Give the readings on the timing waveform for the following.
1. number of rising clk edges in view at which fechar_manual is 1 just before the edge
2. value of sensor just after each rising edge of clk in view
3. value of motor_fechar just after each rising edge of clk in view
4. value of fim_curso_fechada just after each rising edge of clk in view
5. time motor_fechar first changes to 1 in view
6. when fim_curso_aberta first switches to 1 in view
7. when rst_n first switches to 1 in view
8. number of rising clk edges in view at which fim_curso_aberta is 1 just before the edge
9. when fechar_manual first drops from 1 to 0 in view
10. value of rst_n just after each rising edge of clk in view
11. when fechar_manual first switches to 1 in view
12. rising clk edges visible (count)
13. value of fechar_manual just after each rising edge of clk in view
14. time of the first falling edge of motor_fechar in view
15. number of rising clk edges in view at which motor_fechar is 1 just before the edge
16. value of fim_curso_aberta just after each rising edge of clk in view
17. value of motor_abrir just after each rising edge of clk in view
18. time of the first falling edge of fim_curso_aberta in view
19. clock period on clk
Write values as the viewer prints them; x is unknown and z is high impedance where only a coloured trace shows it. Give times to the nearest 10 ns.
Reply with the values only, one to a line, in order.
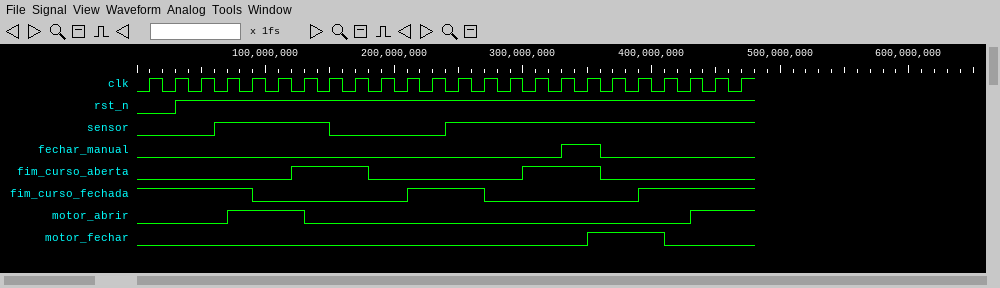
1
0 0 0 1 1 1 1 0 0 0 0 0 1 1 1 1 1 1 1 1 1 1 1 1
0 0 0 0 0 0 0 0 0 0 0 0 0 0 0 0 0 1 1 1 0 0 0 0
1 1 1 1 0 0 0 0 0 0 1 1 1 0 0 0 0 0 0 1 1 1 1 1
350 ns
120 ns
30 ns
6
360 ns
0 1 1 1 1 1 1 1 1 1 1 1 1 1 1 1 1 1 1 1 1 1 1 1
330 ns
24
0 0 0 0 0 0 0 0 0 0 0 0 0 0 0 0 1 1 0 0 0 0 0 0
410 ns
3
0 0 0 0 0 0 1 1 1 0 0 0 0 0 0 1 1 1 0 0 0 0 0 0
0 0 0 1 1 1 0 0 0 0 0 0 0 0 0 0 0 0 0 0 0 1 1 1
180 ns
20 ns
